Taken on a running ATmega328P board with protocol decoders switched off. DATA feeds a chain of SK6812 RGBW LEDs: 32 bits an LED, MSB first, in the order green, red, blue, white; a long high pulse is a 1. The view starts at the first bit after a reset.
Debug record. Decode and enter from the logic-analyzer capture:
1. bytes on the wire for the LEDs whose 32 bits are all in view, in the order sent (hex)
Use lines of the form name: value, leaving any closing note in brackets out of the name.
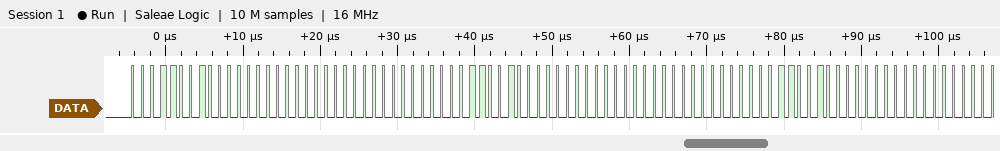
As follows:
bytes on the wire for the LEDs whose 32 bits are all in view, in the order sent: 19 00 00 00 19 00 00 00
